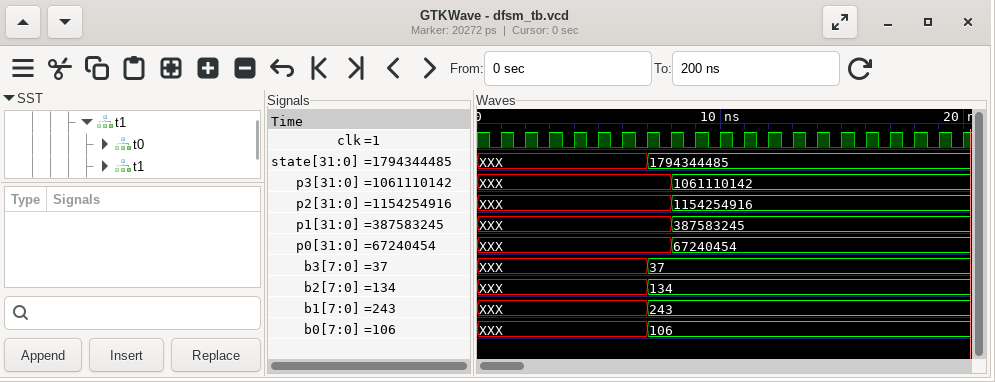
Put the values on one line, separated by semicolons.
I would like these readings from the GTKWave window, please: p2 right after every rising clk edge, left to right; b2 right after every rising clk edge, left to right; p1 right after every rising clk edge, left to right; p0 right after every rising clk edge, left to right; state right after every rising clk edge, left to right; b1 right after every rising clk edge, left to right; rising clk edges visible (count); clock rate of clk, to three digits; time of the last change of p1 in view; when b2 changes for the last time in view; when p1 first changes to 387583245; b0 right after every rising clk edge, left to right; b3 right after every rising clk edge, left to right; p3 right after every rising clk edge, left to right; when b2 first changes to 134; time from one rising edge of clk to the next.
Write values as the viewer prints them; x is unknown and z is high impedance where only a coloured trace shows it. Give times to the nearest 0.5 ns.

XXX, XXX, XXX, XXX, XXX, XXX, XXX, 1154254916, 1154254916, 1154254916, 1154254916, 1154254916, 1154254916, 1154254916, 1154254916, 1154254916, 1154254916, 1154254916, 1154254916, 1154254916; XXX, XXX, XXX, XXX, XXX, XXX, 134, 134, 134, 134, 134, 134, 134, 134, 134, 134, 134, 134, 134, 134; XXX, XXX, XXX, XXX, XXX, XXX, XXX, 387583245, 387583245, 387583245, 387583245, 387583245, 387583245, 387583245, 387583245, 387583245, 387583245, 387583245, 387583245, 387583245; XXX, XXX, XXX, XXX, XXX, XXX, XXX, 67240454, 67240454, 67240454, 67240454, 67240454, 67240454, 67240454, 67240454, 67240454, 67240454, 67240454, 67240454, 67240454; XXX, XXX, XXX, XXX, XXX, XXX, 1794344485, 1794344485, 1794344485, 1794344485, 1794344485, 1794344485, 1794344485, 1794344485, 1794344485, 1794344485, 1794344485, 1794344485, 1794344485, 1794344485; XXX, XXX, XXX, XXX, XXX, XXX, 243, 243, 243, 243, 243, 243, 243, 243, 243, 243, 243, 243, 243, 243; 20; 1.00 GHz; 8 ns; 7 ns; 8 ns; XXX, XXX, XXX, XXX, XXX, XXX, 106, 106, 106, 106, 106, 106, 106, 106, 106, 106, 106, 106, 106, 106; XXX, XXX, XXX, XXX, XXX, XXX, 37, 37, 37, 37, 37, 37, 37, 37, 37, 37, 37, 37, 37, 37; XXX, XXX, XXX, XXX, XXX, XXX, XXX, 1061110142, 1061110142, 1061110142, 1061110142, 1061110142, 1061110142, 1061110142, 1061110142, 1061110142, 1061110142, 1061110142, 1061110142, 1061110142; 7 ns; 1 ns
